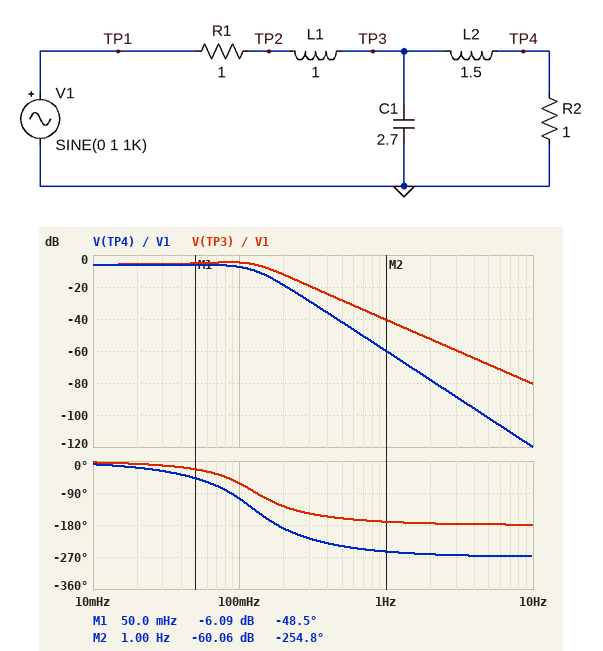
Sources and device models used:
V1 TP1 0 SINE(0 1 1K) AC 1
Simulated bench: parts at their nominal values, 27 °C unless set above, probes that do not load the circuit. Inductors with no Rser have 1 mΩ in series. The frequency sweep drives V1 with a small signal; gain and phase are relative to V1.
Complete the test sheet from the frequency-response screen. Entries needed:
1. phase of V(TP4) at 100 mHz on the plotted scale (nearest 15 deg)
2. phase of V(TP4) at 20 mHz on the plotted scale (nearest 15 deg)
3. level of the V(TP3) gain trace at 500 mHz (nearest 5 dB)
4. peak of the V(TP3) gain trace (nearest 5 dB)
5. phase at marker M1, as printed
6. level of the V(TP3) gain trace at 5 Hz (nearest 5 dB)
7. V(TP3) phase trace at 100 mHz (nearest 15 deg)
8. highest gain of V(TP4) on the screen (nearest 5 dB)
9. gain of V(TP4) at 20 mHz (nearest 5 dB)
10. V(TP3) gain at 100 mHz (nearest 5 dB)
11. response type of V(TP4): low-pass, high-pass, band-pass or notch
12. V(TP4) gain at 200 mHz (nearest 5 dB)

-105 deg
-15 deg
-30 dB
-5 dB
-48.5 deg
-70 dB
-60 deg
-5 dB
-5 dB
-5 dB
low-pass
-20 dB
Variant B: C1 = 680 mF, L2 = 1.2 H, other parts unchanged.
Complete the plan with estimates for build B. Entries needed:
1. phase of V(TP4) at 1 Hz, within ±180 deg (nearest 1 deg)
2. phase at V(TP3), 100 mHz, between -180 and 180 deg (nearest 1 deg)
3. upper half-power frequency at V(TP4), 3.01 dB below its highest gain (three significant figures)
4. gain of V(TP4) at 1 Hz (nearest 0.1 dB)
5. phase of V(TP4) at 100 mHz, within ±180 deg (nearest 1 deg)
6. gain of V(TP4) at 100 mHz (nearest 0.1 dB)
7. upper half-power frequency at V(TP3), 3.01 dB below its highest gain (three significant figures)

107 deg
-12 deg
285 mHz
-45.7 dB
-49 deg
-6.6 dB
308 mHz
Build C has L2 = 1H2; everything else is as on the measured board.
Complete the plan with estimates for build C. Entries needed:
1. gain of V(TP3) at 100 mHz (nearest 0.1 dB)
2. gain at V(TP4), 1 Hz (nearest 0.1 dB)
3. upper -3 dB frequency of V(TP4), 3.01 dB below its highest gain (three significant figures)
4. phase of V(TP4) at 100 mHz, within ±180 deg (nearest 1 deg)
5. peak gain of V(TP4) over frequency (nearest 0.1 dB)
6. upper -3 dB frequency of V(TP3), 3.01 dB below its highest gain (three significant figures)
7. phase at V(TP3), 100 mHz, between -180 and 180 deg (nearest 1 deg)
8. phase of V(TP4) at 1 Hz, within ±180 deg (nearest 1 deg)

-5.3 dB
-58.1 dB
125 mHz
-99 deg
-6.0 dB
152 mHz
-62 deg
107 deg
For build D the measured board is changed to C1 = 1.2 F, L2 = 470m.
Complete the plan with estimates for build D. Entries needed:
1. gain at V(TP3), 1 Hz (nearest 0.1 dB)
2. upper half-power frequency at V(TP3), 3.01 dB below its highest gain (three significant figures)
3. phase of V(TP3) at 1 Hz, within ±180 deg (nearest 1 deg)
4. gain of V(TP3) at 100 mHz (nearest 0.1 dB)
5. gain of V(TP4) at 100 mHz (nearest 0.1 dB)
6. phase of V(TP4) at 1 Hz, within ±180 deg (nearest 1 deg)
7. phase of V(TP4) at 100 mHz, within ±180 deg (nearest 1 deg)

-33.1 dB
265 mHz
-170 deg
-5.7 dB
-6.1 dB
119 deg
-50 deg
